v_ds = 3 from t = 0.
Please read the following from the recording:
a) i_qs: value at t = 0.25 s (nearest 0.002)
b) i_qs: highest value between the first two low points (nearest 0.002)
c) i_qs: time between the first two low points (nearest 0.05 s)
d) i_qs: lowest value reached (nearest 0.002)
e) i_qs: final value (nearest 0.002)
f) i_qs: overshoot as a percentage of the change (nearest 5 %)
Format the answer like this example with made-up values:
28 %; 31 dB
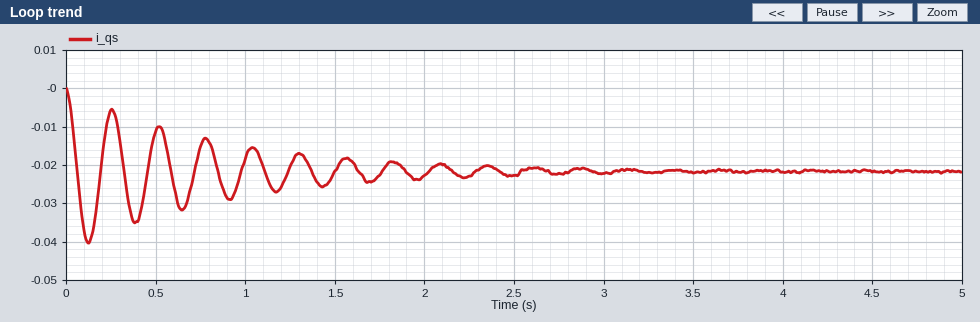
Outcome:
-0.006; -0.006; 0.25 s; -0.040; -0.022; 85 %
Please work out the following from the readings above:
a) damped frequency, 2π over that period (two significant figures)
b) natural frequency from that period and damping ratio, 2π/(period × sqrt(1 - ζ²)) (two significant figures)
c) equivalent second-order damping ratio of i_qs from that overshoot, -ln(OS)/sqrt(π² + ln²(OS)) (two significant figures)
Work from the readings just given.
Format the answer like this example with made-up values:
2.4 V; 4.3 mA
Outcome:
25 rad/s; 25 rad/s; 0.052
